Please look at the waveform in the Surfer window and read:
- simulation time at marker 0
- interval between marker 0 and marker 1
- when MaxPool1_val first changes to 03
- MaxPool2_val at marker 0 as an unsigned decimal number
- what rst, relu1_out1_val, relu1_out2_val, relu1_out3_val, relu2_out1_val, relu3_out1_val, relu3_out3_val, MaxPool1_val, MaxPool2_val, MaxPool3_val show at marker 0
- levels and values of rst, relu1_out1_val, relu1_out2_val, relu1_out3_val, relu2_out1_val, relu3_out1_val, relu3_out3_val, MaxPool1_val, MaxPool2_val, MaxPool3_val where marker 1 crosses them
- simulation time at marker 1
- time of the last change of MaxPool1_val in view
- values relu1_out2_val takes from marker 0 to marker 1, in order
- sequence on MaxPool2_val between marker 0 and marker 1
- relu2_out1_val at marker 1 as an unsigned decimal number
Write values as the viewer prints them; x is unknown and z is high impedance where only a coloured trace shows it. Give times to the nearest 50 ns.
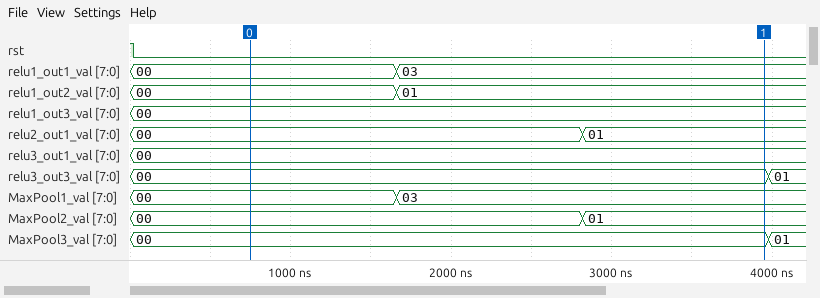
750 ns
3200 ns
1650 ns
0
rst=0, relu1_out1_val=00, relu1_out2_val=00, relu1_out3_val=00, relu2_out1_val=00, relu3_out1_val=00, relu3_out3_val=00, MaxPool1_val=00, MaxPool2_val=00, MaxPool3_val=00
rst=0, relu1_out1_val=03, relu1_out2_val=01, relu1_out3_val=00, relu2_out1_val=01, relu3_out1_val=00, relu3_out3_val=00, MaxPool1_val=03, MaxPool2_val=01, MaxPool3_val=00
3950 ns
1650 ns
00, 01
00, 01
1
